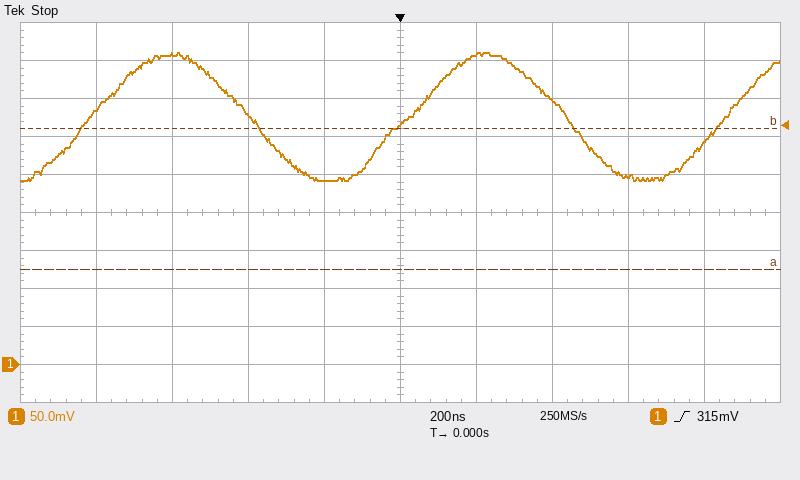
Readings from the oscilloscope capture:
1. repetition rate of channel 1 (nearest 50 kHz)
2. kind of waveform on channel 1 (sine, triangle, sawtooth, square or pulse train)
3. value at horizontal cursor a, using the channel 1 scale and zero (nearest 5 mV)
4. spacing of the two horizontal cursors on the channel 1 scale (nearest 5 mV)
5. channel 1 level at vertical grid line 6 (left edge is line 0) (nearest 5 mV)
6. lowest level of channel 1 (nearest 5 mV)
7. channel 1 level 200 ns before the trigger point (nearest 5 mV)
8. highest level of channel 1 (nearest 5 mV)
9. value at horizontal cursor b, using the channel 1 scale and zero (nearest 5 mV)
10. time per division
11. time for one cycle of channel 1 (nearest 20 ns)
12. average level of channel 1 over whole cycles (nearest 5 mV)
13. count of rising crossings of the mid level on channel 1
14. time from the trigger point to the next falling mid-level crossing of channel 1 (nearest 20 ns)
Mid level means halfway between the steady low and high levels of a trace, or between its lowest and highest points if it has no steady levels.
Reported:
1.20 MHz
sine
125 mV
185 mV
410 mV
240 mV
240 mV
410 mV
310 mV
200 ns
840 ns
325 mV
3
440 ns
